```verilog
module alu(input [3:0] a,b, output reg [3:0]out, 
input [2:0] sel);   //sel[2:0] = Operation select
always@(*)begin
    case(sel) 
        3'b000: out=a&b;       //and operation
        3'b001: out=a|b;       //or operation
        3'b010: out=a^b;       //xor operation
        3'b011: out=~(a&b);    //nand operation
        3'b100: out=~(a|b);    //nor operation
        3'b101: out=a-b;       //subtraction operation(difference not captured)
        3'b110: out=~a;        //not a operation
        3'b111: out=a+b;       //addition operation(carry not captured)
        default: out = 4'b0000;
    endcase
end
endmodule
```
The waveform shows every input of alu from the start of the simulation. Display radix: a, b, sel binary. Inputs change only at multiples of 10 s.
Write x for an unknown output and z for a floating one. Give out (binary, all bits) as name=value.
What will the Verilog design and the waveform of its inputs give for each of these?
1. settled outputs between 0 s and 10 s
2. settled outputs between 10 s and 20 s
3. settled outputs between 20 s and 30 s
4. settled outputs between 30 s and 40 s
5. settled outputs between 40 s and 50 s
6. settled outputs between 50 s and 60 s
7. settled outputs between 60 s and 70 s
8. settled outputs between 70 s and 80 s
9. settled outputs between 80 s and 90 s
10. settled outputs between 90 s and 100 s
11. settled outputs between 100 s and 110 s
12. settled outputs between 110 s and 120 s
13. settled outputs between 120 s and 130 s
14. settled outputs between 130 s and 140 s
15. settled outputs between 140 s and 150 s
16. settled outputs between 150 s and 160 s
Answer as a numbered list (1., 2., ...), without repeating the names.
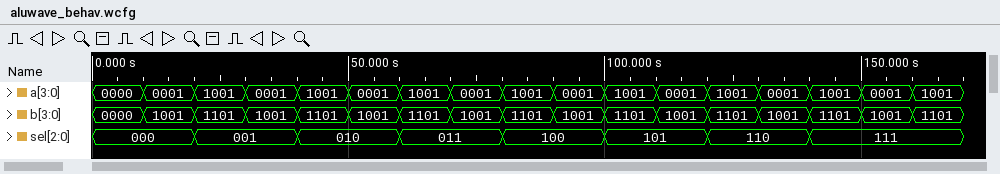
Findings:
1. out=0000
2. out=0001
3. out=1101
4. out=1001
5. out=0100
6. out=1000
7. out=0110
8. out=1110
9. out=0010
10. out=0110
11. out=1100
12. out=1000
13. out=0110
14. out=1110
15. out=0110
16. out=1010
